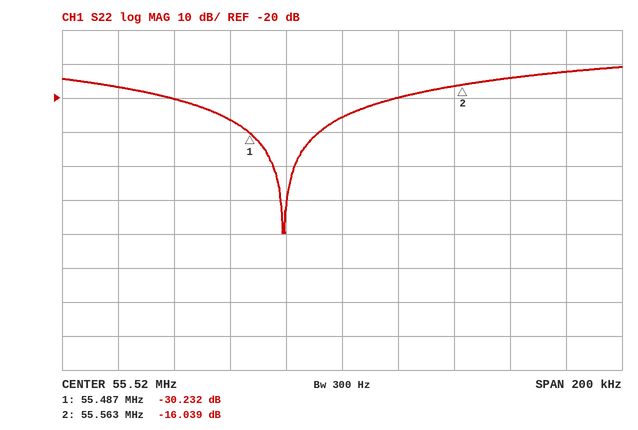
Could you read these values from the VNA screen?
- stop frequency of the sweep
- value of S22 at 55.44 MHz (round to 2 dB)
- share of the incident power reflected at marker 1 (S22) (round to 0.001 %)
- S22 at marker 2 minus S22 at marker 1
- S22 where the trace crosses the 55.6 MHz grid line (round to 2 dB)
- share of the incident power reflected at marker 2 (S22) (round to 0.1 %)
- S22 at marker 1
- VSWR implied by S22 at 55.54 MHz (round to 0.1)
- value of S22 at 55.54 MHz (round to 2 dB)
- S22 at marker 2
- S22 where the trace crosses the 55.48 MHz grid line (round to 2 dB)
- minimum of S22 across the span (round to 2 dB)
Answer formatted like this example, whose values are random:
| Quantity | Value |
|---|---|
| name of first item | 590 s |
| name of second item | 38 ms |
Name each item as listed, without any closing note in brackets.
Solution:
| Quantity | Value |
|---|---|
| stop frequency of the sweep | 55.62 MHz |
| value of S22 at 55.44 MHz | -16 dB |
| share of the incident power reflected at marker 1 (S22) | 0.095 % |
| S22 at marker 2 minus S22 at marker 1 | 14.193 dB |
| S22 where the trace crosses the 55.6 MHz grid line | -12 dB |
| share of the incident power reflected at marker 2 (S22) | 2.5 % |
| S22 at marker 1 | -30.232 dB |
| VSWR implied by S22 at 55.54 MHz | 1.2 |
| value of S22 at 55.54 MHz | -20 dB |
| S22 at marker 2 | -16.039 dB |
| S22 where the trace crosses the 55.48 MHz grid line | -26 dB |
| minimum of S22 across the span | -60 dB |
